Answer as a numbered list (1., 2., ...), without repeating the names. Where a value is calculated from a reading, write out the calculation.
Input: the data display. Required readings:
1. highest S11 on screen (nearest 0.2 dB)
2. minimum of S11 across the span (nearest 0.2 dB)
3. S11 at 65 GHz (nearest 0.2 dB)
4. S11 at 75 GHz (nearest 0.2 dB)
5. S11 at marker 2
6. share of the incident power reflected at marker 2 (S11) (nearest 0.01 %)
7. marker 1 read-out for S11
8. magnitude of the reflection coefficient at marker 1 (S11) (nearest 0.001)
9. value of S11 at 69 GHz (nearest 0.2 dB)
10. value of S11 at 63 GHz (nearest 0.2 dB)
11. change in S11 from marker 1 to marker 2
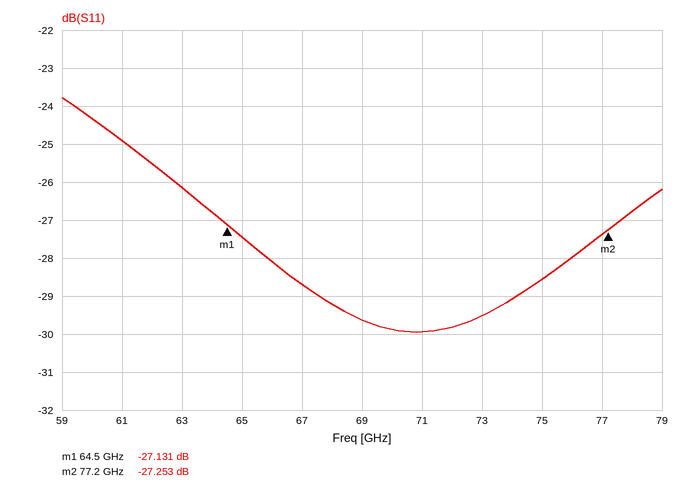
1. -23.8 dB
2. -30.0 dB
3. -27.4 dB
4. -28.6 dB
5. -27.253 dB
6. 10^(-27.253/10) ≈ 0.19 %
7. -27.131 dB
8. 10^(-27.131/20) ≈ 0.044
9. -29.6 dB
10. -26.2 dB
11. -27.253 − (-27.131) = -0.122 dB
